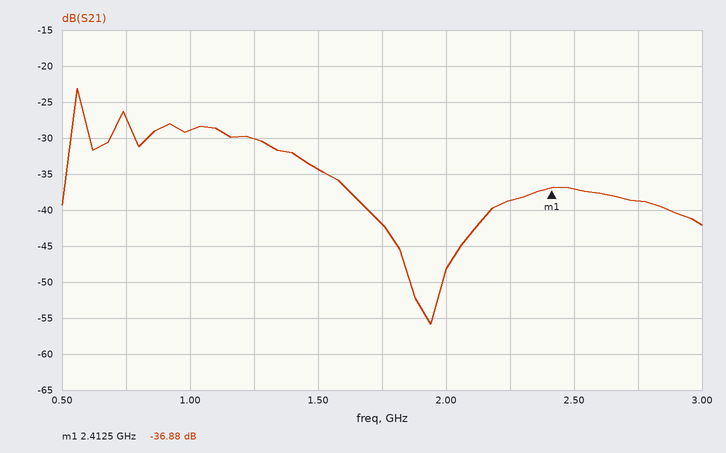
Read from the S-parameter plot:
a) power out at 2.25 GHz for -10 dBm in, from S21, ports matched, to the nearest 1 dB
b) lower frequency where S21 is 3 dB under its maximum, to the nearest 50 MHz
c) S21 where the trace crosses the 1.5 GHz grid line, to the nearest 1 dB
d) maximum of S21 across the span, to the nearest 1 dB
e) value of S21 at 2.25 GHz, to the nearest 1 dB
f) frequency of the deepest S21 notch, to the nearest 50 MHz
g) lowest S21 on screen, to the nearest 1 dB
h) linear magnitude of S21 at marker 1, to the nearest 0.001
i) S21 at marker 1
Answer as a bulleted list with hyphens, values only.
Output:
- -49 dBm
- 550 MHz
- -34 dB
- -23 dB
- -39 dB
- 1.95 GHz
- -56 dB
- 0.014
- -36.88 dB
